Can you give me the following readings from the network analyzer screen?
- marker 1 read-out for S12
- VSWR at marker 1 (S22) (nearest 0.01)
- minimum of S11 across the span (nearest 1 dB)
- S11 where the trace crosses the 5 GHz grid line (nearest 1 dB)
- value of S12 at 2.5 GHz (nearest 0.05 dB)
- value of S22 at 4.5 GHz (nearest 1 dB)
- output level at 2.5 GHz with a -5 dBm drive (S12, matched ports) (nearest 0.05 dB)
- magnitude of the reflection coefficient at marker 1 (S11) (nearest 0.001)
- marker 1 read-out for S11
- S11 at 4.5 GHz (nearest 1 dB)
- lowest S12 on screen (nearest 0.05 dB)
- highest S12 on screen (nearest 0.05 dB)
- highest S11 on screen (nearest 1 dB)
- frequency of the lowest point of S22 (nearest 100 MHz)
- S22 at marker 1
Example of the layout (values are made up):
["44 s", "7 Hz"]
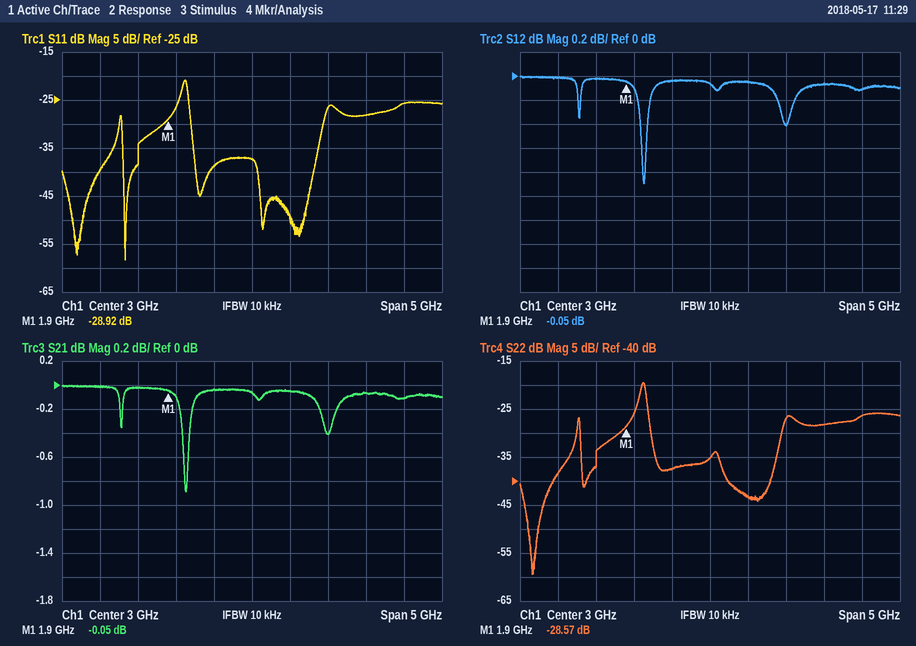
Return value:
["-0.05 dB", "1.08", "-58 dB", "-26 dB", "-0.05 dB", "-28 dB", "-5.05 dBm", "0.036", "-28.92 dB", "-28 dB", "-0.90 dB", "0.00 dB", "-21 dB", "700 MHz", "-28.57 dB"]
